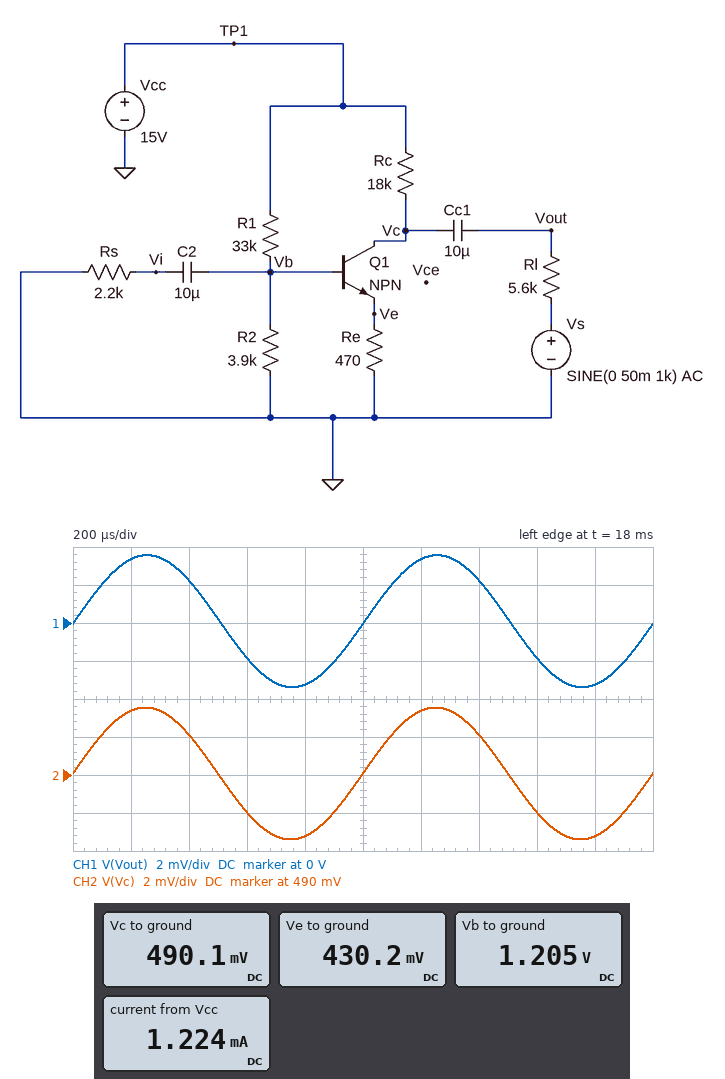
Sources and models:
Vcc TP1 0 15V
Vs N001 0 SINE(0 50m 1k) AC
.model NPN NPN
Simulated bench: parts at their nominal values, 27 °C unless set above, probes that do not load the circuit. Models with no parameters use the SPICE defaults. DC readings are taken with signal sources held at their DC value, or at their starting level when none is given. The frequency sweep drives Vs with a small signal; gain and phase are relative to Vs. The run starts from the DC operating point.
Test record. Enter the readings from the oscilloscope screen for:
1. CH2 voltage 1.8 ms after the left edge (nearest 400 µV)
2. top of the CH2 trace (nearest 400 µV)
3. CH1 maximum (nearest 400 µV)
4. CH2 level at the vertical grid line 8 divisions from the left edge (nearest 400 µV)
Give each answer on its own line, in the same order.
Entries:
486.8 mV
493.6 mV
3.6 mV
488.0 mV
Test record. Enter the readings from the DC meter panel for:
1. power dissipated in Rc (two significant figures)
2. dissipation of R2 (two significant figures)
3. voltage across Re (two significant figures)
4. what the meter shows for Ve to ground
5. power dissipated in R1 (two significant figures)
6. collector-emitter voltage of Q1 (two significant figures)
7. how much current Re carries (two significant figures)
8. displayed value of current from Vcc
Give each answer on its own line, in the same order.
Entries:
12 mW
370 µW
430 mV
430.2 mV
5.8 mW
60 mV
920 µA
1.224 mA
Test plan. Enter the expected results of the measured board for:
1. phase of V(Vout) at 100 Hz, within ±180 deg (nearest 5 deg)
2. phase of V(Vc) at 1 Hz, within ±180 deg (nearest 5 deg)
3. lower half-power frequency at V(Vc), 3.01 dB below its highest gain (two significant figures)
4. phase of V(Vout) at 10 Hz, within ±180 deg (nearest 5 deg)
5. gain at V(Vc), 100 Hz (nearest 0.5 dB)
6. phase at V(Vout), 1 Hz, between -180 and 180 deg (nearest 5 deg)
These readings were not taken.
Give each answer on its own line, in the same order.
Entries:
-20 deg
70 deg
2.3 Hz
-60 deg
-23.0 dB
-20 deg
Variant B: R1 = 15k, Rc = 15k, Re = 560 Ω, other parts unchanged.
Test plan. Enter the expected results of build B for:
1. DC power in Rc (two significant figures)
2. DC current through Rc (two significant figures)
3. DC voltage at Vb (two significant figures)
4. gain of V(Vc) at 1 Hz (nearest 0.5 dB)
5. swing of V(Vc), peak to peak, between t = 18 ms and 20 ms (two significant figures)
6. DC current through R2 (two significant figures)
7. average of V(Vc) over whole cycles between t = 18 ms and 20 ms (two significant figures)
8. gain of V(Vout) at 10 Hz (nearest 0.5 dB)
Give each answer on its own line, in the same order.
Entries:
13 mW
940 µA
1.6 V
-31.0 dB
6.7 mV
410 µA
840 mV
-11.5 dB
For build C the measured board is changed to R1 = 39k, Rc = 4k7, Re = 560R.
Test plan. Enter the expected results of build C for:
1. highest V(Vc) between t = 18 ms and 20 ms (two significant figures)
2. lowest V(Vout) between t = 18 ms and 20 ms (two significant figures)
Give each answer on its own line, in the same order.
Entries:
10 V
-23 mV
